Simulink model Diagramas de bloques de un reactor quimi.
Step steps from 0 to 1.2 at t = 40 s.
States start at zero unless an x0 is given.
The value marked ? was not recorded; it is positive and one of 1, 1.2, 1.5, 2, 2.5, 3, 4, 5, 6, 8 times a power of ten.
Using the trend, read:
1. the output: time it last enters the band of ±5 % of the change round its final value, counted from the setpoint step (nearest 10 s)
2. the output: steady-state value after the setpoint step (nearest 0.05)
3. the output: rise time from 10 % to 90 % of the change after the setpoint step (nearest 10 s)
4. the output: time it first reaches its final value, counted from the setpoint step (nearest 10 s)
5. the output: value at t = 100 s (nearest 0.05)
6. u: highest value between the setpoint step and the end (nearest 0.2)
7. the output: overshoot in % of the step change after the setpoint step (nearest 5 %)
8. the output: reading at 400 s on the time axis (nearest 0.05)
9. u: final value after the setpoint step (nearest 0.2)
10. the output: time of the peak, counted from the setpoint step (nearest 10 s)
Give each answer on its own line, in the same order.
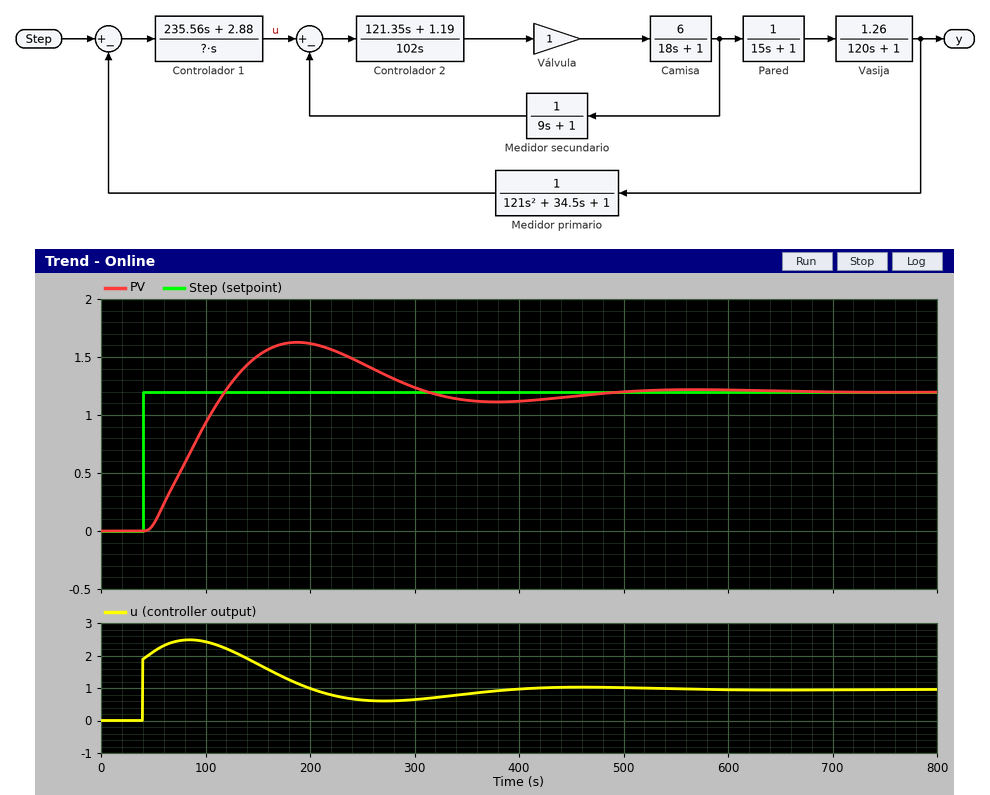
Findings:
390 s
1.20
60 s
80 s
0.95
2.4
35 %
1.10
1.0
150 s
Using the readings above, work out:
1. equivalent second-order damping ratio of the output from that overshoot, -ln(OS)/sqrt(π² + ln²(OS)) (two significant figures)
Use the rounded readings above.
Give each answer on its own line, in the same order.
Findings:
0.32
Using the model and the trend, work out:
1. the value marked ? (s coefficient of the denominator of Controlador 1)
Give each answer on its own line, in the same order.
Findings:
150
